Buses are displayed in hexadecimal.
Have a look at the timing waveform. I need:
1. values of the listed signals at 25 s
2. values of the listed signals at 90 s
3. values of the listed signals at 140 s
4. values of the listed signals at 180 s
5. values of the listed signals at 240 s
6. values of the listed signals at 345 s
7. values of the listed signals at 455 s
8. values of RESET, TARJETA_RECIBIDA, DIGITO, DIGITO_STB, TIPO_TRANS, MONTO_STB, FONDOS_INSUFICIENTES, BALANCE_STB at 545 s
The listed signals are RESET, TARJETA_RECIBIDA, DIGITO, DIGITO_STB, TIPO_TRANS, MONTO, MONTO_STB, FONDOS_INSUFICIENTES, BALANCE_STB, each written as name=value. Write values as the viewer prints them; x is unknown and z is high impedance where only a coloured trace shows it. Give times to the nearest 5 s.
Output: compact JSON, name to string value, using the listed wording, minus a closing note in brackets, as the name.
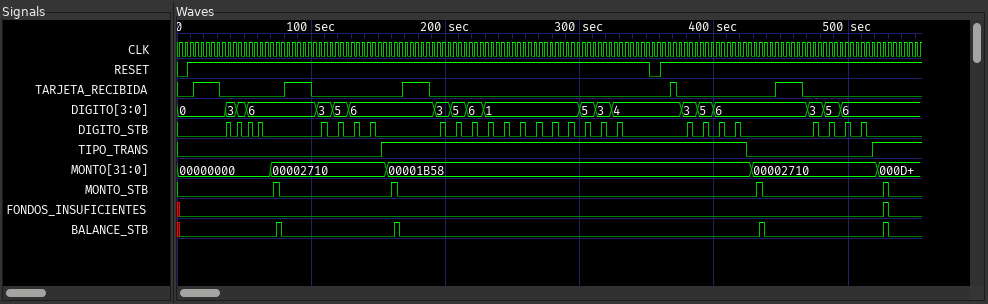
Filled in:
{"values of the listed signals at 25 s": "RESET=1, TARJETA_RECIBIDA=1, DIGITO=0, DIGITO_STB=0, TIPO_TRANS=0, MONTO=00000000, MONTO_STB=0, FONDOS_INSUFICIENTES=0, BALANCE_STB=0", "values of the listed signals at 90 s": "RESET=1, TARJETA_RECIBIDA=1, DIGITO=6, DIGITO_STB=0, TIPO_TRANS=0, MONTO=00002710, MONTO_STB=0, FONDOS_INSUFICIENTES=0, BALANCE_STB=0", "values of the listed signals at 140 s": "RESET=1, TARJETA_RECIBIDA=0, DIGITO=6, DIGITO_STB=0, TIPO_TRANS=0, MONTO=00002710, MONTO_STB=0, FONDOS_INSUFICIENTES=0, BALANCE_STB=0", "values of the listed signals at 180 s": "RESET=1, TARJETA_RECIBIDA=1, DIGITO=6, DIGITO_STB=0, TIPO_TRANS=1, MONTO=00001B58, MONTO_STB=0, FONDOS_INSUFICIENTES=0, BALANCE_STB=0", "values of the listed signals at 240 s": "RESET=1, TARJETA_RECIBIDA=0, DIGITO=1, DIGITO_STB=0, TIPO_TRANS=1, MONTO=00001B58, MONTO_STB=0, FONDOS_INSUFICIENTES=0, BALANCE_STB=0", "values of the listed signals at 345 s": "RESET=1, TARJETA_RECIBIDA=0, DIGITO=4, DIGITO_STB=0, TIPO_TRANS=1, MONTO=00001B58, MONTO_STB=0, FONDOS_INSUFICIENTES=0, BALANCE_STB=0", "values of the listed signals at 455 s": "RESET=1, TARJETA_RECIBIDA=1, DIGITO=6, DIGITO_STB=0, TIPO_TRANS=0, MONTO=00002710, MONTO_STB=0, FONDOS_INSUFICIENTES=0, BALANCE_STB=0", "values of RESET, TARJETA_RECIBIDA, DIGITO, DIGITO_STB, TIPO_TRANS, MONTO_STB, FONDOS_INSUFICIENTES, BALANCE_STB at 545 s": "RESET=1, TARJETA_RECIBIDA=0, DIGITO=6, DIGITO_STB=0, TIPO_TRANS=1, MONTO_STB=0, FONDOS_INSUFICIENTES=0, BALANCE_STB=0"}
